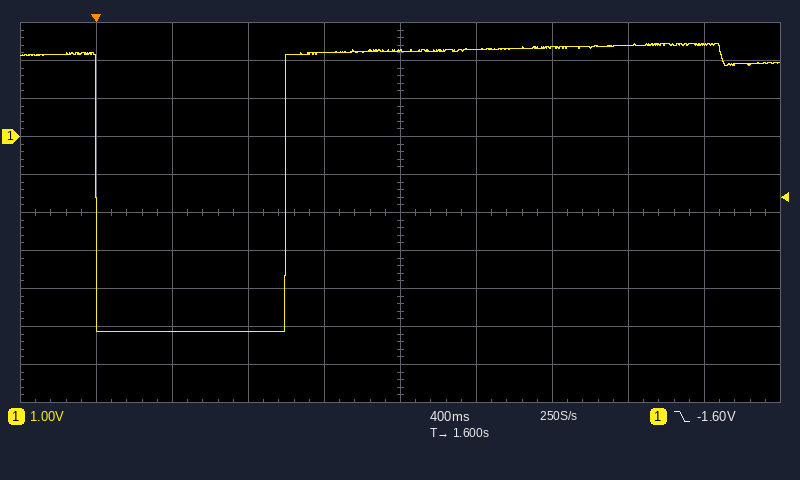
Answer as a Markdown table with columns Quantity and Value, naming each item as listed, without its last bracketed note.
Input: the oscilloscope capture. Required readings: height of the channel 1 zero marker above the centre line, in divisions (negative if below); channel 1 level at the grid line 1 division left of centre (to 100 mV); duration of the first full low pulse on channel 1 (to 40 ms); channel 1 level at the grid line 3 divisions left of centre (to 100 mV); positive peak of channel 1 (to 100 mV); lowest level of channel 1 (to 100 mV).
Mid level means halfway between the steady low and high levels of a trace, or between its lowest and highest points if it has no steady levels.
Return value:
| Quantity | Value |
|---|---|
| height of the channel 1 zero marker above the centre line, in divisions | +2.0 div |
| channel 1 level at the grid line 1 division left of centre | 2.2 V |
| duration of the first full low pulse on channel 1 | 1.00 s |
| channel 1 level at the grid line 3 divisions left of centre | -5.1 V |
| positive peak of channel 1 | 2.4 V |
| lowest level of channel 1 | -5.1 V |
